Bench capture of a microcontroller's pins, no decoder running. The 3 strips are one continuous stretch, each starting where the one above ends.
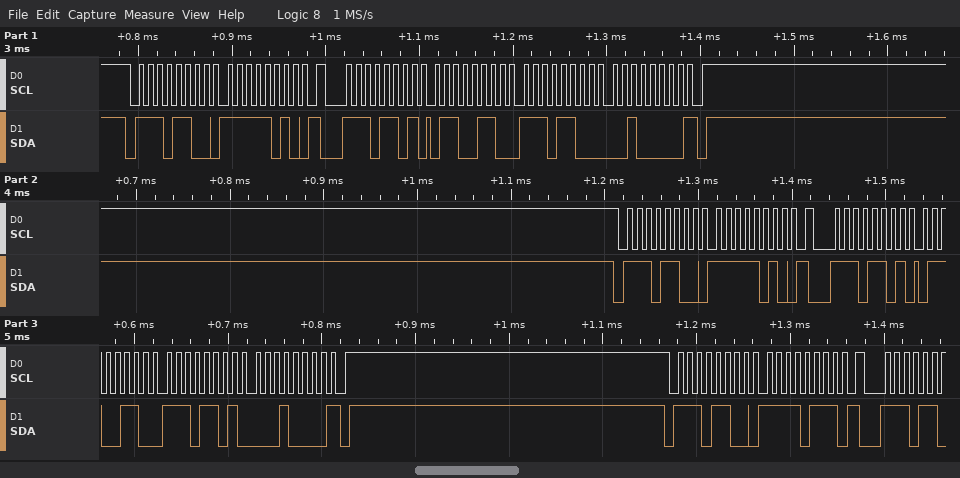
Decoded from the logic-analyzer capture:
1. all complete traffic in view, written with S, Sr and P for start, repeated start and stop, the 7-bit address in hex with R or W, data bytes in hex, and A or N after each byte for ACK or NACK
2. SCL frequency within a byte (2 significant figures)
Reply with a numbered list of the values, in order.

1. S 76W A FA A Sr 76R A 66 A EC A 20 N P S 76W A FA A Sr 76R A 66 A ED A 10 N P S 76W A F7 A
2. 100 kHz
